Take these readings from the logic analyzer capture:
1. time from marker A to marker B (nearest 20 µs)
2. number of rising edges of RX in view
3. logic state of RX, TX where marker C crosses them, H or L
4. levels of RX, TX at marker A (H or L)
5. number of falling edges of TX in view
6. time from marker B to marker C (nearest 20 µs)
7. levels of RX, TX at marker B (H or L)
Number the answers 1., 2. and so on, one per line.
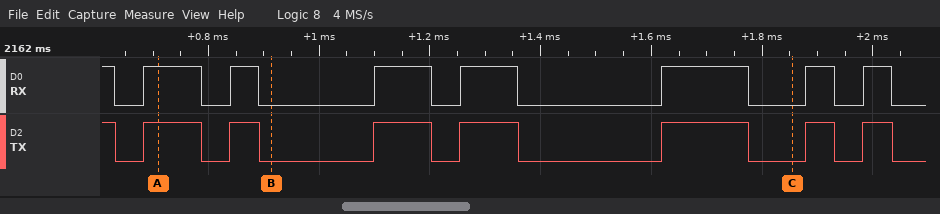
1. 200 µs
2. 7
3. RX=L, TX=L
4. RX=H, TX=H
5. 8
6. 940 µs
7. RX=L, TX=L
